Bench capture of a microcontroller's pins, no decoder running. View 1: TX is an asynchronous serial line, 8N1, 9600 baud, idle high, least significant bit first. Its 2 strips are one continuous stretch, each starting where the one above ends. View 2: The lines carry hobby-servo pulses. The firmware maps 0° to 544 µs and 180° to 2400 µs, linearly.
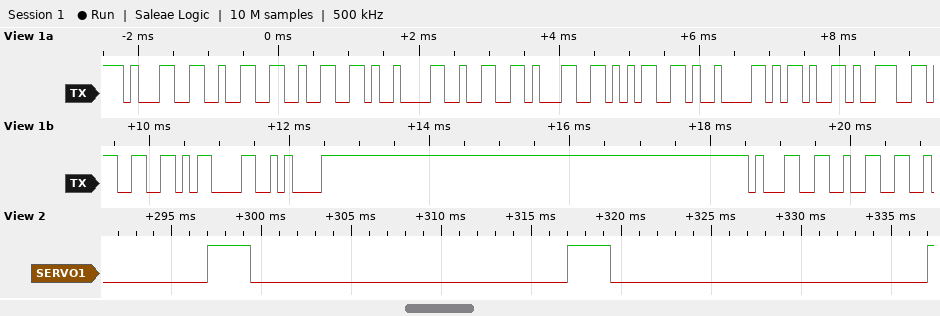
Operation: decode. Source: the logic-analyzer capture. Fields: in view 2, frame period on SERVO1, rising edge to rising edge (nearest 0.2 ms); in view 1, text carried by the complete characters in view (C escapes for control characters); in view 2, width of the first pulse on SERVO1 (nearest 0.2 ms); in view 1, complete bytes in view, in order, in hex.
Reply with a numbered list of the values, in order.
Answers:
1. 20.0 ms
2. "122\t215\t-93\r\n12"
3. 2.4 ms
4. 31 32 32 09 32 31 35 09 2D 39 33 0D 0A 31 32
